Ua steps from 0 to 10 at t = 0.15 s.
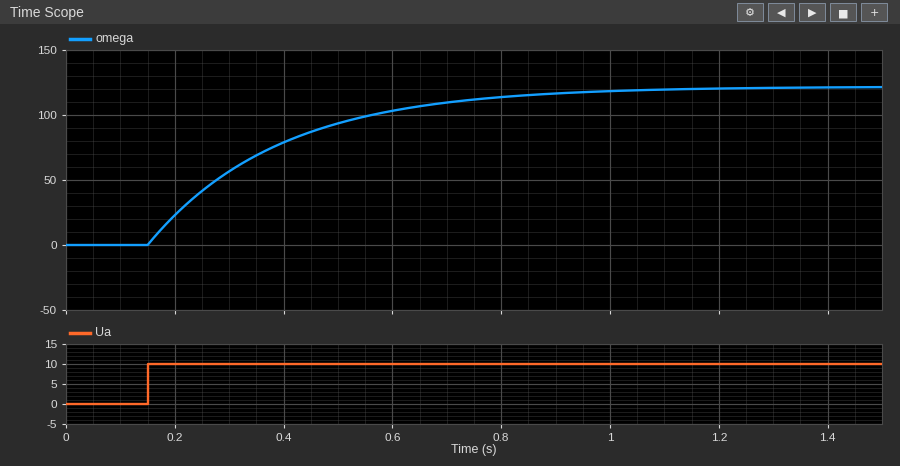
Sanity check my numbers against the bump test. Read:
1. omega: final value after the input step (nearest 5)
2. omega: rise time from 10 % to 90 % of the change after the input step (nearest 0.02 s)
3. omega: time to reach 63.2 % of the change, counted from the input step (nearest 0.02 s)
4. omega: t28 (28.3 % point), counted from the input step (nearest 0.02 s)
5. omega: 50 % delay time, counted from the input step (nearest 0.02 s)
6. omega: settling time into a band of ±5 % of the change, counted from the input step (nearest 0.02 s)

120
0.52 s
0.24 s
0.08 s
0.16 s
0.72 s
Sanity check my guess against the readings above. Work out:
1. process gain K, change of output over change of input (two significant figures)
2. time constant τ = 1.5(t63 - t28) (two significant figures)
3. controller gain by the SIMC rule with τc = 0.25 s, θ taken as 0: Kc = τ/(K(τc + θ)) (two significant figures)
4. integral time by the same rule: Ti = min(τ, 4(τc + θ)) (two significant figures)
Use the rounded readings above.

12
0.24 s
0.080
0.24 s
